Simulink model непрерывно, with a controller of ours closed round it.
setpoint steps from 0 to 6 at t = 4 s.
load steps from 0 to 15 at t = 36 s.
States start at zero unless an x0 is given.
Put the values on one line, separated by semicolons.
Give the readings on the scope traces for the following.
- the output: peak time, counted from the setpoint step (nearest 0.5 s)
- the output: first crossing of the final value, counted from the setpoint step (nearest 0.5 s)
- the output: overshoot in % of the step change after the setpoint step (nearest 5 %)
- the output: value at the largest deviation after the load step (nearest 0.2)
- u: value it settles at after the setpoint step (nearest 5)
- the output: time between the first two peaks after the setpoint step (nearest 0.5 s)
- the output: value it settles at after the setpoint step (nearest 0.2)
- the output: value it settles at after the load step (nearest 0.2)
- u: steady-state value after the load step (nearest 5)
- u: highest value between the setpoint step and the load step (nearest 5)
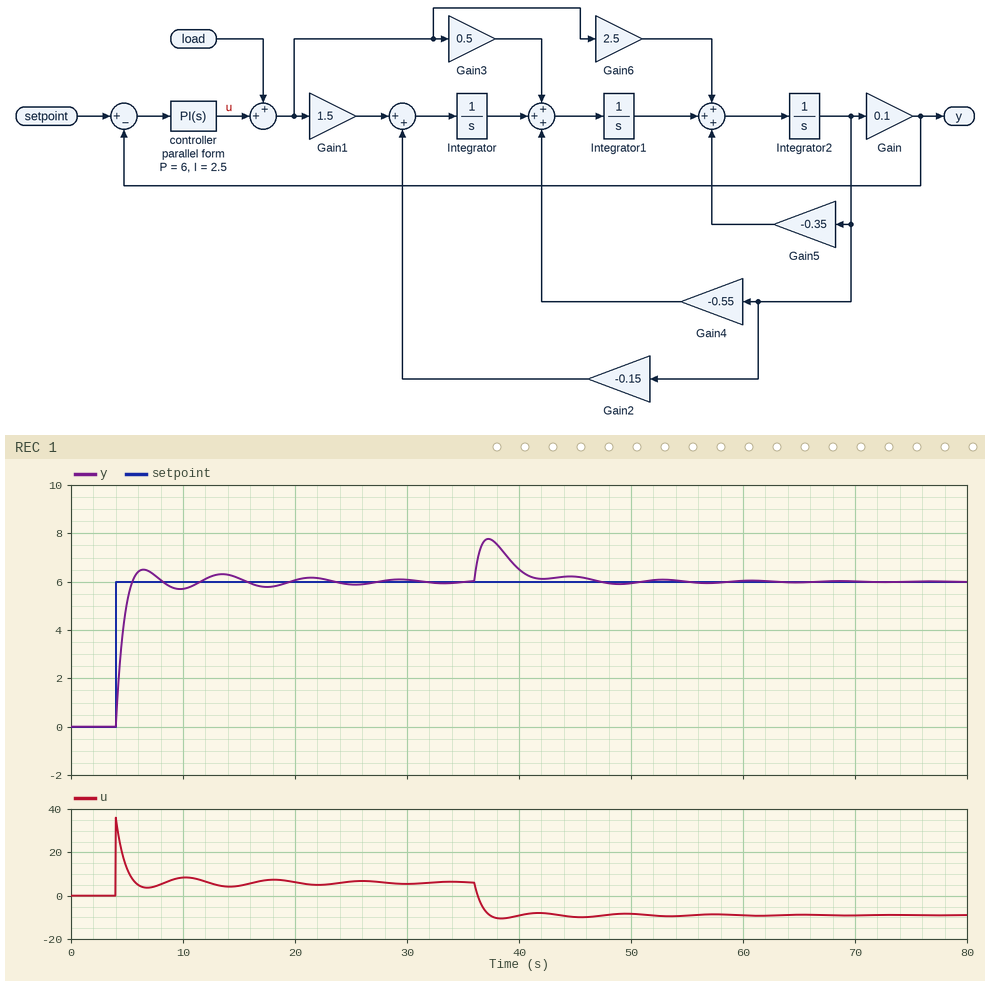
2.5 s; 1.5 s; 10 %; 7.8; 5; 7.0 s; 6.0; 6.0; -10; 35
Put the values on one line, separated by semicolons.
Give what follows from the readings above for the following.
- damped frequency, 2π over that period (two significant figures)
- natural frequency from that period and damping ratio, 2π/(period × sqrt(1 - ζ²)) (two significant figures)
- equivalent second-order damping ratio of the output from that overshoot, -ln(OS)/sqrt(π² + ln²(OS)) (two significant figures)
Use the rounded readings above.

0.90 rad/s; 1.1 rad/s; 0.59
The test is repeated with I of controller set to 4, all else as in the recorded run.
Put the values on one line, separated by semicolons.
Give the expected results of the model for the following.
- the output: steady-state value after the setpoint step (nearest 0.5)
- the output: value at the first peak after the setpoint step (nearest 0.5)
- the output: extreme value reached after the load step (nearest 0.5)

6.0; 7.0; 7.5
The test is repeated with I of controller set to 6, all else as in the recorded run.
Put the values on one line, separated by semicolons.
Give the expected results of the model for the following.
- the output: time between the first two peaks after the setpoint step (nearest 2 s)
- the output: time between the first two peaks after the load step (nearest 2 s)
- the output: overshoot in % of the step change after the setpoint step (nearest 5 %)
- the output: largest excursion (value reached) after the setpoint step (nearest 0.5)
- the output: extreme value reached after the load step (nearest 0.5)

6 s; 6 s; 20 %; 7.0; 7.5
